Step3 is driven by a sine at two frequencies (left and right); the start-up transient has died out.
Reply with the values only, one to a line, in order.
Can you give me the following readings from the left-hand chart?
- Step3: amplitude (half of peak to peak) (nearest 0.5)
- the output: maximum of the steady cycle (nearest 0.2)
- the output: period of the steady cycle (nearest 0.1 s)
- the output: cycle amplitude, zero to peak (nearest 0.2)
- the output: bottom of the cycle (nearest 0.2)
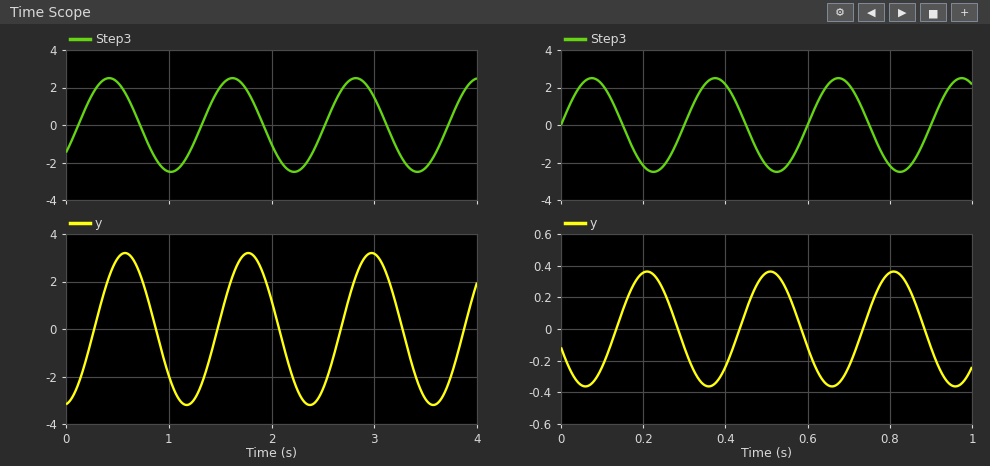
2.5
3.2
1.2 s
3.2
-3.2
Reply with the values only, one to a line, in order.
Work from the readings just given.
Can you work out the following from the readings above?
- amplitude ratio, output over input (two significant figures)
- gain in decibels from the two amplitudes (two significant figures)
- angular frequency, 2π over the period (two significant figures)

1.3
2.1 dB
5.2 rad/s
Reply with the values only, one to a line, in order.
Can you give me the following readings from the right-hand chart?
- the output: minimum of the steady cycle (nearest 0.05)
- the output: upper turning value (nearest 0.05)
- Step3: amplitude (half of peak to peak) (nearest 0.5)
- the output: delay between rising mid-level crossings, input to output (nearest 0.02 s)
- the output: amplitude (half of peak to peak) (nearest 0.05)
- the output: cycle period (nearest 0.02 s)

-0.35
0.35
2.5
0.14 s
0.35
0.30 s
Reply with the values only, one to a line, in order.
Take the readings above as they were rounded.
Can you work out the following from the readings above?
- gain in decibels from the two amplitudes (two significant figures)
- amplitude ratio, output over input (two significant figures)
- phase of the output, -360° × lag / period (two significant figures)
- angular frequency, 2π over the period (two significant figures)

-17 dB
0.14
-170°
21 rad/s
